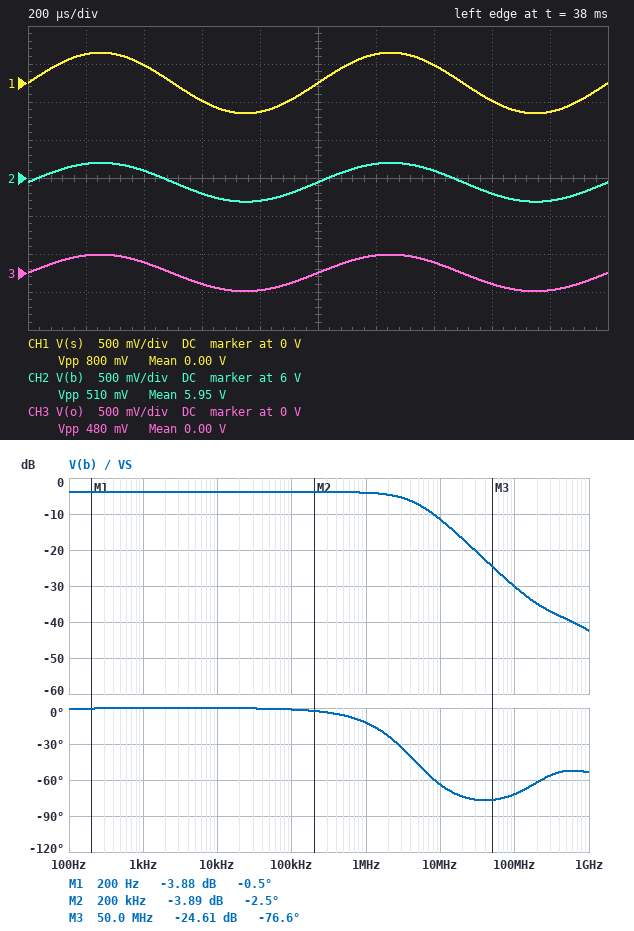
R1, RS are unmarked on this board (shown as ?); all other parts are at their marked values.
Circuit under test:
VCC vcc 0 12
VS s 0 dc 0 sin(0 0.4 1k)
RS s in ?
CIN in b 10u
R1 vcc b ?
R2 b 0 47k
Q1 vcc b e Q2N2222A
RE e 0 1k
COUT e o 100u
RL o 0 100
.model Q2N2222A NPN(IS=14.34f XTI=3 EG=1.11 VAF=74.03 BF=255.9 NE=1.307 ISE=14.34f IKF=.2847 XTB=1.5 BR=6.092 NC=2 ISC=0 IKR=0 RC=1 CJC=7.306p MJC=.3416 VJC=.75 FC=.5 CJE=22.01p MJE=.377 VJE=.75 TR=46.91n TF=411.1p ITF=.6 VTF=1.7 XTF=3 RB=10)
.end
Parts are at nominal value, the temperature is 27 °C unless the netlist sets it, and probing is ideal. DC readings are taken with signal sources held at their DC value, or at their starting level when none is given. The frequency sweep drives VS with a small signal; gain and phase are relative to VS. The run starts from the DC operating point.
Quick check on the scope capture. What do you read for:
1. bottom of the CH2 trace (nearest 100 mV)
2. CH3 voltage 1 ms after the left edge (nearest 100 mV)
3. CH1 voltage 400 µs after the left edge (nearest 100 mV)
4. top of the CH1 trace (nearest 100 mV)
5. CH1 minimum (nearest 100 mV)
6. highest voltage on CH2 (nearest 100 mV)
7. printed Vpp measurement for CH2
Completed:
5.7 V
0 V
200 mV
400 mV
-400 mV
6.2 V
510 mV
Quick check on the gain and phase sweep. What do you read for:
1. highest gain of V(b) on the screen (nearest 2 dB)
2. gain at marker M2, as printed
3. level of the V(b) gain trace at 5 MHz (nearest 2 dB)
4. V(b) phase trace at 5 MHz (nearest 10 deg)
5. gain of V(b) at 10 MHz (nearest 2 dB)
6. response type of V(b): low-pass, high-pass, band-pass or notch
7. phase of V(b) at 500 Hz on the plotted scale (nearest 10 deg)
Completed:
-4 dB
-3.89 dB
-8 dB
-50 deg
-12 dB
low-pass
0 deg
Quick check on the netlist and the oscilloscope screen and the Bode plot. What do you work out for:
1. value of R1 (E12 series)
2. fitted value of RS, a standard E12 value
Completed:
39 kΩ
5.6 kΩ
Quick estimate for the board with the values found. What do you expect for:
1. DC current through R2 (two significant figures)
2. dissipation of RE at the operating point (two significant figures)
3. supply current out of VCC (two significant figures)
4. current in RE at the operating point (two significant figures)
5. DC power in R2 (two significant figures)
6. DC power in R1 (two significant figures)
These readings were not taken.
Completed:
130 µA
28 mW
5.4 mA
5.3 mA
750 µW
940 µW
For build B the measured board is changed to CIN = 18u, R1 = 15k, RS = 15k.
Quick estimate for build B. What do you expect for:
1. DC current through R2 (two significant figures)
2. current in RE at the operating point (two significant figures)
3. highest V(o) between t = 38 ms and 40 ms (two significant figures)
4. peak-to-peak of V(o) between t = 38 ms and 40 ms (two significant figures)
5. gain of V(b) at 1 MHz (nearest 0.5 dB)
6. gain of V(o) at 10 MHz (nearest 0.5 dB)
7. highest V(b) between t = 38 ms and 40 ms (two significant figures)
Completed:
180 µA
7.9 mA
120 mV
240 mV
-10.5 dB
-20.0 dB
8.7 V
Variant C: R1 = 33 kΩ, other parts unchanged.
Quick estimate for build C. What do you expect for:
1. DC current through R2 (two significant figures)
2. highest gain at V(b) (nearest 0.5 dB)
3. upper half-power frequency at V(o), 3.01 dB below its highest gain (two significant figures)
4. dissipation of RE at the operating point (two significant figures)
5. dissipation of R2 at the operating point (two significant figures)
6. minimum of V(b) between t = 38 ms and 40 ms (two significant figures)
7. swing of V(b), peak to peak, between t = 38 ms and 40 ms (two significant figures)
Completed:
140 µA
-3.0 dB
4.6 MHz
33 mW
880 µW
6.2 V
500 mV
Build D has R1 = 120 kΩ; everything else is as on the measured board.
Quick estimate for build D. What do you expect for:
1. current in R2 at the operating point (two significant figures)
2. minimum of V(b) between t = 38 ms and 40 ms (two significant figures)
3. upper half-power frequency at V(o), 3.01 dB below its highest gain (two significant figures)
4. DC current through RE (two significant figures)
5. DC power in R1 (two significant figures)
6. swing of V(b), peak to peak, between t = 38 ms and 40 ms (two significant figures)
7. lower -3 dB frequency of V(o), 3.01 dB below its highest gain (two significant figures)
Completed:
63 µA
2.7 V
3.6 MHz
2.3 mA
680 µW
560 mV
12 Hz
